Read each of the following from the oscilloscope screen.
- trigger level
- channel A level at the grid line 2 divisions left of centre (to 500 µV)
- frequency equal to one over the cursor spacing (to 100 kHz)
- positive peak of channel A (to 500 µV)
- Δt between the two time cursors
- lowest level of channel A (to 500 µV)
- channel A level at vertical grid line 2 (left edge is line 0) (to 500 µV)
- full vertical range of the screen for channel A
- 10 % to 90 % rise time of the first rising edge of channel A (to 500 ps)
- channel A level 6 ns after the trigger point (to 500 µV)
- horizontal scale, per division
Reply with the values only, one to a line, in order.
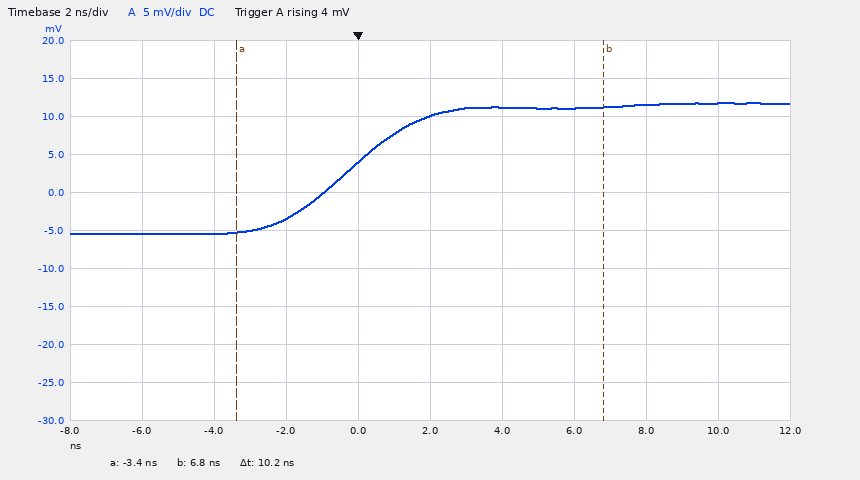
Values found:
4 mV
-3.5 mV
98.0 MHz
12.0 mV
10.2 ns
-5.5 mV
-5.5 mV
50 mV
4.0 ns
11.0 mV
2 ns
